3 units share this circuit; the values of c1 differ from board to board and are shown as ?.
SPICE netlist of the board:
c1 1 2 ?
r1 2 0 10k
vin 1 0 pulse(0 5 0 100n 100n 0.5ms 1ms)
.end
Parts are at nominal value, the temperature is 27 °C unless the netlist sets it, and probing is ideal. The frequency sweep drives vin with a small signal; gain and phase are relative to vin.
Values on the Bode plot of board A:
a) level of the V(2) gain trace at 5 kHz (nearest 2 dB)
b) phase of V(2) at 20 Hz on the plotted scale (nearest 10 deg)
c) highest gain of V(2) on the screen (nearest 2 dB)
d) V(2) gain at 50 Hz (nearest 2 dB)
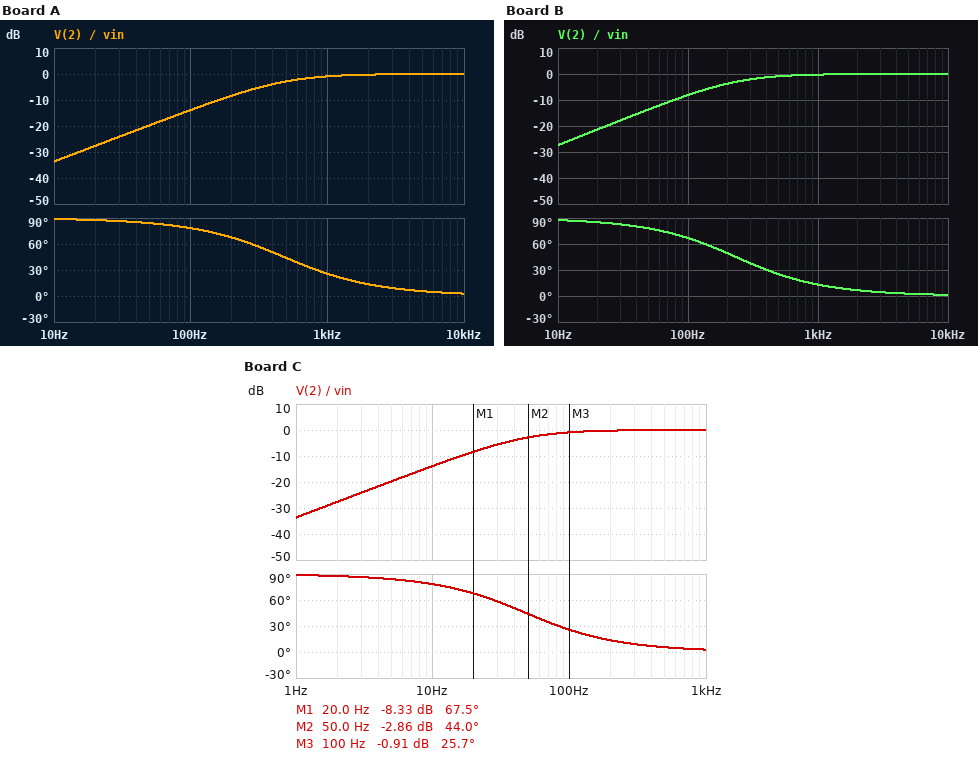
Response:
0 dB
90 deg
0 dB
-20 dB
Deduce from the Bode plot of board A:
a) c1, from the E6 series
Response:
33 nF
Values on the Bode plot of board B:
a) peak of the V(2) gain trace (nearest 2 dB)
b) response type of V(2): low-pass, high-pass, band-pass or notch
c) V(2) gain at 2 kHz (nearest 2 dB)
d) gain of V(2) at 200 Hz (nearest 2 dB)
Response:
0 dB
high-pass
0 dB
-4 dB
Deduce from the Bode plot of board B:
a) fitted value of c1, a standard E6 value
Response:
68 nF
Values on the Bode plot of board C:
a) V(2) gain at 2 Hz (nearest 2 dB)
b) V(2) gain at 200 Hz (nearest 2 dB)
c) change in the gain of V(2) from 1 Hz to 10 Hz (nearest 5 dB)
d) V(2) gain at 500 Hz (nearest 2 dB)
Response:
-28 dB
0 dB
20 dB
0 dB
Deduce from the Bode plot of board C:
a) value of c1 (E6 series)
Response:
330 nF
